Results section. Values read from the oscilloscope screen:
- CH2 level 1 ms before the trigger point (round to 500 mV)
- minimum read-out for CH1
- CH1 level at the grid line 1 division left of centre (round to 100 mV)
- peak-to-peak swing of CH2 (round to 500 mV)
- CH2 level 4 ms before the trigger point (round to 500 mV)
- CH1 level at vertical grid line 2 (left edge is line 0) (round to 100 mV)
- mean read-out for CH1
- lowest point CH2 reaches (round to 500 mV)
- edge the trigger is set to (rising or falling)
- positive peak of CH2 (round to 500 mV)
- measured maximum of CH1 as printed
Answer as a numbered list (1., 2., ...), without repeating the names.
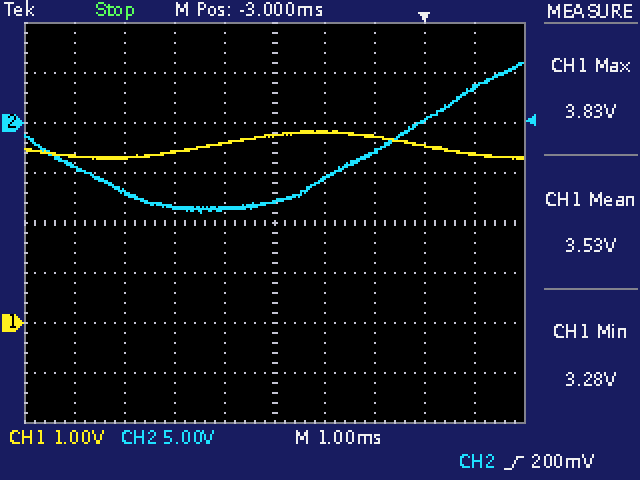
1. -3.0 V
2. 3.28 V
3. 3.6 V
4. 15.0 V
5. -8.5 V
6. 3.3 V
7. 3.53 V
8. -9.0 V
9. rising
10. 6.0 V
11. 3.83 V
